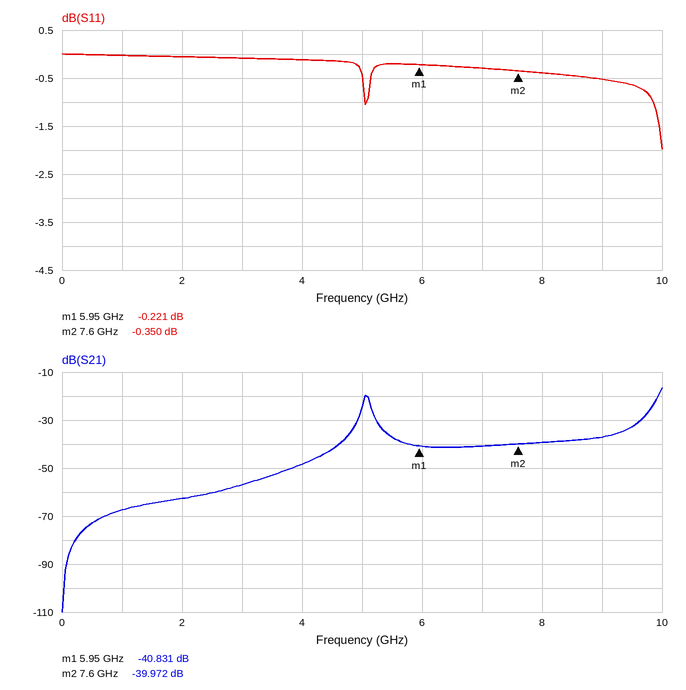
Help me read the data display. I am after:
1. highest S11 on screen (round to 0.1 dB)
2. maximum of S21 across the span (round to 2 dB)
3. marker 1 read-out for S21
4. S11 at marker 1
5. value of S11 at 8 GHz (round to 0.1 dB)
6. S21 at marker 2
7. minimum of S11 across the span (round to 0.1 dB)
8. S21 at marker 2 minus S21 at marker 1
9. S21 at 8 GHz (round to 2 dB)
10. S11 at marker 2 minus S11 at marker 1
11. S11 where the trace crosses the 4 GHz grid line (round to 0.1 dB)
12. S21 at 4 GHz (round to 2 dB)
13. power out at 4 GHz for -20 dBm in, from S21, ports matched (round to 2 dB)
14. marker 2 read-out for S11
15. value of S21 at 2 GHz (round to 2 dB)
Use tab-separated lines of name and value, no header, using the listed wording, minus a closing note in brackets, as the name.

highest S11 on screen	0.0 dB
maximum of S21 across the span	-16 dB
marker 1 read-out for S21	-40.831 dB
S11 at marker 1	-0.221 dB
value of S11 at 8 GHz	-0.4 dB
S21 at marker 2	-39.972 dB
minimum of S11 across the span	-2.0 dB
S21 at marker 2 minus S21 at marker 1	0.859 dB
S21 at 8 GHz	-40 dB
S11 at marker 2 minus S11 at marker 1	-0.129 dB
S11 where the trace crosses the 4 GHz grid line	-0.1 dB
S21 at 4 GHz	-48 dB
power out at 4 GHz for -20 dBm in, from S21, ports matched	-68 dBm
marker 2 read-out for S11	-0.350 dB
value of S21 at 2 GHz	-62 dB
